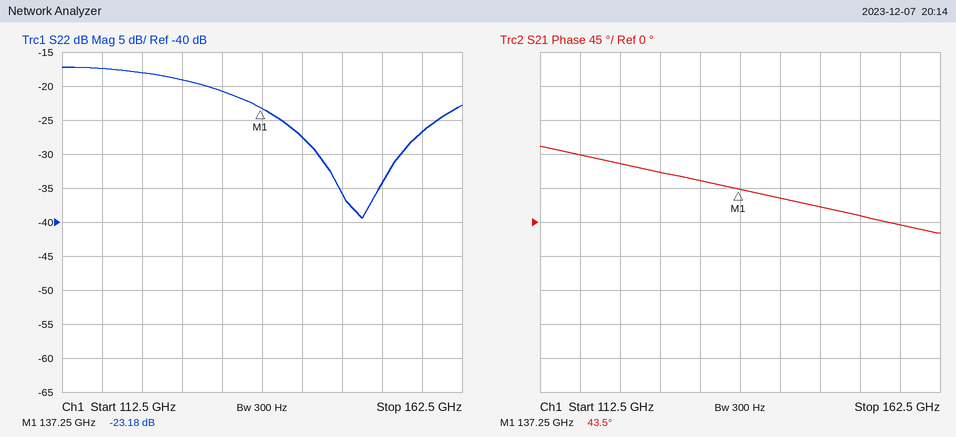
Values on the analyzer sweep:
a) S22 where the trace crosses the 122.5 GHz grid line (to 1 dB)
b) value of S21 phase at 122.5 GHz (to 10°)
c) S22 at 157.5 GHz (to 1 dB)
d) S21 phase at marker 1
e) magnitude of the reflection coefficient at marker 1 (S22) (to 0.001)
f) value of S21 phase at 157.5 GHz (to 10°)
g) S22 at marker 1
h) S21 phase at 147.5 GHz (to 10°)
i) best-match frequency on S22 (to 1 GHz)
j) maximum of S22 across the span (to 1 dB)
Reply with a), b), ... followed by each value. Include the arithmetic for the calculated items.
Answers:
a) -18 dB
b) 80°
c) -27 dB
d) 43.5°
e) 10^(-23.18/20) ≈ 0.069
f) 0°
g) -23.18 dB
h) 20°
i) 150 GHz
j) -17 dB
